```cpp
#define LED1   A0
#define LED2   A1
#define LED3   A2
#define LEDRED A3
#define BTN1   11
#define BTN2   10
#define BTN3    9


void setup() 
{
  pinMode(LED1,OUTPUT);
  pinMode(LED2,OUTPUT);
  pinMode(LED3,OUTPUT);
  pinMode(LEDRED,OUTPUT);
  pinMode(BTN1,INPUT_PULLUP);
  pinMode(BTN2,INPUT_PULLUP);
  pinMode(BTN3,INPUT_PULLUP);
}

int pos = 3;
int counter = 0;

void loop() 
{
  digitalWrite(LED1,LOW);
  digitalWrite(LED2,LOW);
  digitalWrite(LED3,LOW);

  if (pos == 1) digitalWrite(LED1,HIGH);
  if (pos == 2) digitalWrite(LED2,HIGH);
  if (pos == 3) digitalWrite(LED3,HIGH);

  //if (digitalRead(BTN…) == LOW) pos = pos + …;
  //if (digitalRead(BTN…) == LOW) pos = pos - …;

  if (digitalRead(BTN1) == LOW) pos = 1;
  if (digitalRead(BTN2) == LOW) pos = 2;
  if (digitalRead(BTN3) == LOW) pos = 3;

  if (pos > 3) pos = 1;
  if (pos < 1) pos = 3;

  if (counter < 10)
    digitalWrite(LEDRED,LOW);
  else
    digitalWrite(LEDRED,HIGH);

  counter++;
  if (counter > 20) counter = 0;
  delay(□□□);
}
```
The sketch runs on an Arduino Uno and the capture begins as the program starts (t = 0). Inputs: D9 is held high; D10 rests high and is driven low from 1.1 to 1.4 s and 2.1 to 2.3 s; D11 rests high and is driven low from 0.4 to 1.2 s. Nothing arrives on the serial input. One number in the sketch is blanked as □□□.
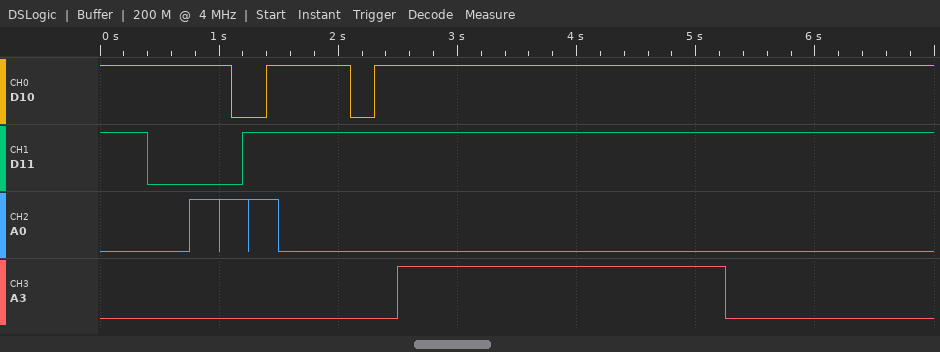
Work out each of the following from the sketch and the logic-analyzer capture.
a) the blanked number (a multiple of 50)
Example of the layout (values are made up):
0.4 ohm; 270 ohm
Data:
250
